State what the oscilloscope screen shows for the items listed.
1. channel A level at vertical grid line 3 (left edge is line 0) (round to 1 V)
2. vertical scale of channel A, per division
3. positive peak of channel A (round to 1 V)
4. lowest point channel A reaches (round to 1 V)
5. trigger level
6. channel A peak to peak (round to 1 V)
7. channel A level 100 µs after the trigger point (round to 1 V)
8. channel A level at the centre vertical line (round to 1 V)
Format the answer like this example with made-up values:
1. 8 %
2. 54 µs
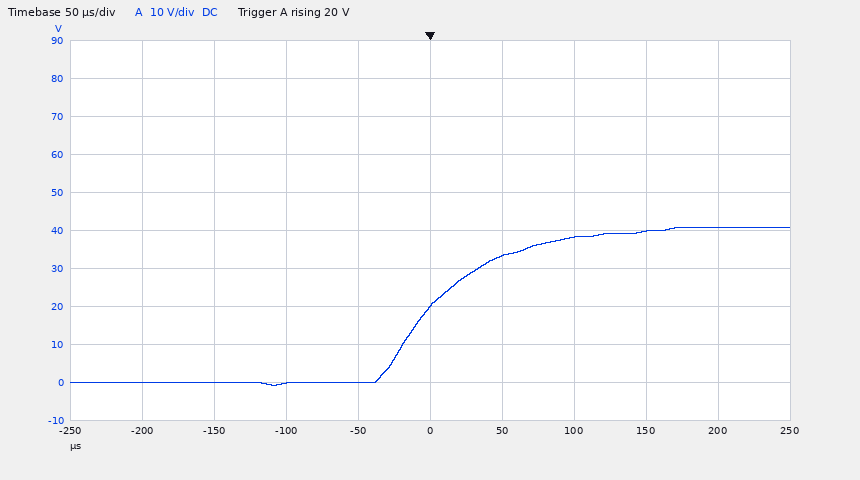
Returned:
1. 0 V
2. 10 V
3. 41 V
4. -1 V
5. 20 V
6. 42 V
7. 38 V
8. 20 V
